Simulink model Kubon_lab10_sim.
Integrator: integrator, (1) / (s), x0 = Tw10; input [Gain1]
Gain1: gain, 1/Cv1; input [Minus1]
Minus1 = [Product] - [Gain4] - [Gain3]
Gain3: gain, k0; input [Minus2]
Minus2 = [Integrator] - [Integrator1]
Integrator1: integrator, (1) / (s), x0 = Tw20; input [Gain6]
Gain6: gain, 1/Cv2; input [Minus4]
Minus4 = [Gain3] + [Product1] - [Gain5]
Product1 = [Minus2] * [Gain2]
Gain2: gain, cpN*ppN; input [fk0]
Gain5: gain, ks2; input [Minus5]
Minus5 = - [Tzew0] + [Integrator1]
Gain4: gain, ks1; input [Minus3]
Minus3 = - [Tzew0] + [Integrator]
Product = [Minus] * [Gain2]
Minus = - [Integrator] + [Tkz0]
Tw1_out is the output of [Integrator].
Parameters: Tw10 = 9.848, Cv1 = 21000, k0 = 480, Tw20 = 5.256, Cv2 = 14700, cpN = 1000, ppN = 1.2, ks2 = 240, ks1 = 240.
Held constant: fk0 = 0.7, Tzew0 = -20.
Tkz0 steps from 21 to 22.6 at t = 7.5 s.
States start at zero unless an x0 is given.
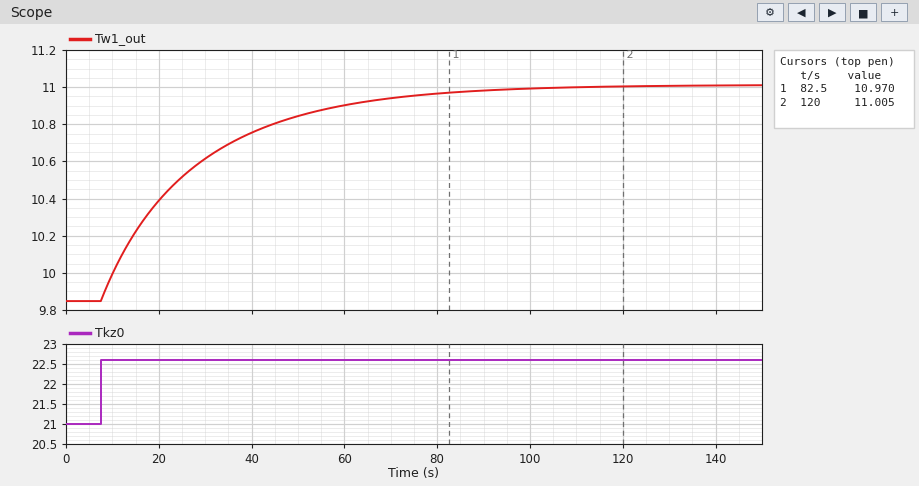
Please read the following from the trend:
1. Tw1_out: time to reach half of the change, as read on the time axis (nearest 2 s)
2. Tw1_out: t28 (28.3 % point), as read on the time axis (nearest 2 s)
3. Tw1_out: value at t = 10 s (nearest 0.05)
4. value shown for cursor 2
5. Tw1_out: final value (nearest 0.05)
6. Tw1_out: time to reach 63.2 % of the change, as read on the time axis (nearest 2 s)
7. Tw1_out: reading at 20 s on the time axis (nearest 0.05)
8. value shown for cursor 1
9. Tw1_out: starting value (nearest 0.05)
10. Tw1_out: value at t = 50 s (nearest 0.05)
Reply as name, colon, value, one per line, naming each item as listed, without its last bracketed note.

Tw1_out: time to reach half of the change, as read on the time axis: 22 s
Tw1_out: t28 (28.3 % point), as read on the time axis: 14 s
Tw1_out: value at t = 10 s: 10.00
value shown for cursor 2: 11.005
Tw1_out: final value: 11.00
Tw1_out: time to reach 63.2 % of the change, as read on the time axis: 28 s
Tw1_out: reading at 20 s on the time axis: 10.40
value shown for cursor 1: 10.970
Tw1_out: starting value: 9.85
Tw1_out: value at t = 50 s: 10.85
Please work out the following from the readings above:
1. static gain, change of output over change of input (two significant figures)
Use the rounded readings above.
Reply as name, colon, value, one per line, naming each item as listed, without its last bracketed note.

static gain, change of output over change of input: 0.72
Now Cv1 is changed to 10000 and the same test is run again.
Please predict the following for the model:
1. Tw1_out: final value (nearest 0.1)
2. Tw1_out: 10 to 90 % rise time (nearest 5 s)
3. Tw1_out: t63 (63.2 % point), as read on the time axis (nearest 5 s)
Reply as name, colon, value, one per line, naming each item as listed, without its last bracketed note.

Tw1_out: final value: 11.0
Tw1_out: 10 to 90 % rise time: 30 s
Tw1_out: t63 (63.2 % point), as read on the time axis: 20 s
